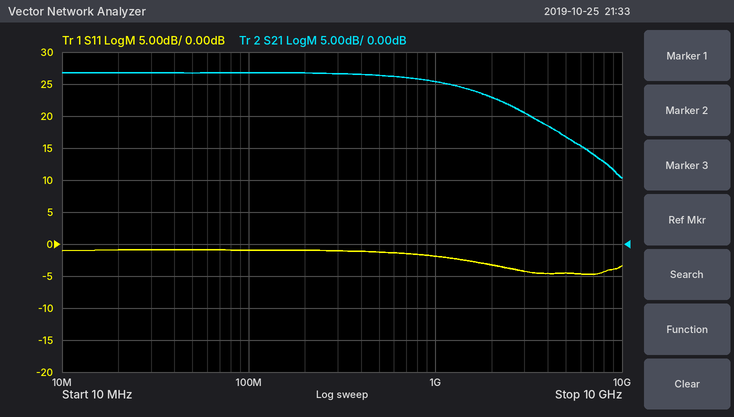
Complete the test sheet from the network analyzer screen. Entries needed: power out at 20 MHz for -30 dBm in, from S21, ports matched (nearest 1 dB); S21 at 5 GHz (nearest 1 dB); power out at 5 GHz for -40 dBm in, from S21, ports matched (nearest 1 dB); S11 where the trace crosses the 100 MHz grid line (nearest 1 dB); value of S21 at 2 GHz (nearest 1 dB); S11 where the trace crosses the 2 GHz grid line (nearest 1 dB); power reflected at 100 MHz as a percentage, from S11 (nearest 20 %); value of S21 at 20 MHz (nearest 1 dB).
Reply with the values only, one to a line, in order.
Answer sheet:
-3 dBm
17 dB
-23 dBm
-1 dB
23 dB
-3 dB
80 %
27 dB
